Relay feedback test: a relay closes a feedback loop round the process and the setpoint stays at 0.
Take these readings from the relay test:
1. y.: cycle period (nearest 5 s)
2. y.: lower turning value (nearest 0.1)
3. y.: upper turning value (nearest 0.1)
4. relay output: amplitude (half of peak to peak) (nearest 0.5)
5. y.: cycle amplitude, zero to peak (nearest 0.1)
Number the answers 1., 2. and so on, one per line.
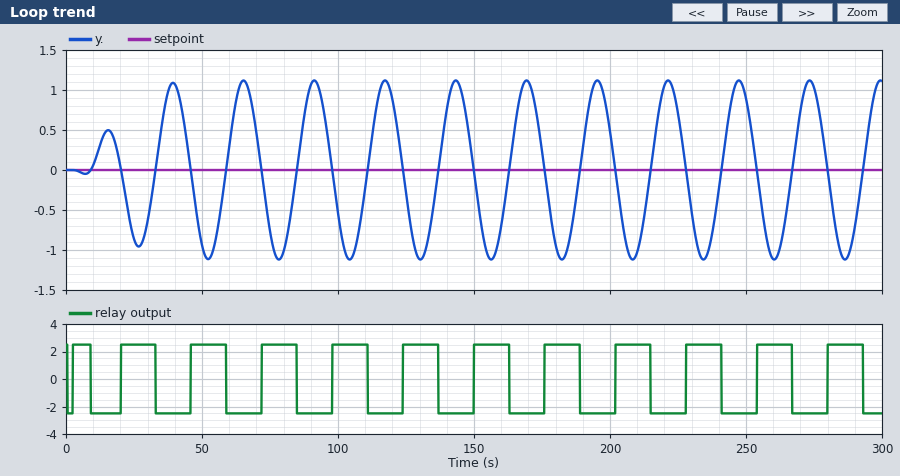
1. 25 s
2. -1.1
3. 1.1
4. 2.5
5. 1.1
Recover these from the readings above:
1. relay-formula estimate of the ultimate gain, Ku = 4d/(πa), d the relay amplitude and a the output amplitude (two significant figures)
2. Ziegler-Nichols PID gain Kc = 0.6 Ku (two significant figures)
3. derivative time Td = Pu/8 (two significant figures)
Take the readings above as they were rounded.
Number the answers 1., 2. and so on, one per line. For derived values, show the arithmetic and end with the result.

1. 4 × 2.5 / (π × 1.1) = 2.9
2. 0.6 × 2.9 = 1.7
3. 25 / 8 = 3.1 s
